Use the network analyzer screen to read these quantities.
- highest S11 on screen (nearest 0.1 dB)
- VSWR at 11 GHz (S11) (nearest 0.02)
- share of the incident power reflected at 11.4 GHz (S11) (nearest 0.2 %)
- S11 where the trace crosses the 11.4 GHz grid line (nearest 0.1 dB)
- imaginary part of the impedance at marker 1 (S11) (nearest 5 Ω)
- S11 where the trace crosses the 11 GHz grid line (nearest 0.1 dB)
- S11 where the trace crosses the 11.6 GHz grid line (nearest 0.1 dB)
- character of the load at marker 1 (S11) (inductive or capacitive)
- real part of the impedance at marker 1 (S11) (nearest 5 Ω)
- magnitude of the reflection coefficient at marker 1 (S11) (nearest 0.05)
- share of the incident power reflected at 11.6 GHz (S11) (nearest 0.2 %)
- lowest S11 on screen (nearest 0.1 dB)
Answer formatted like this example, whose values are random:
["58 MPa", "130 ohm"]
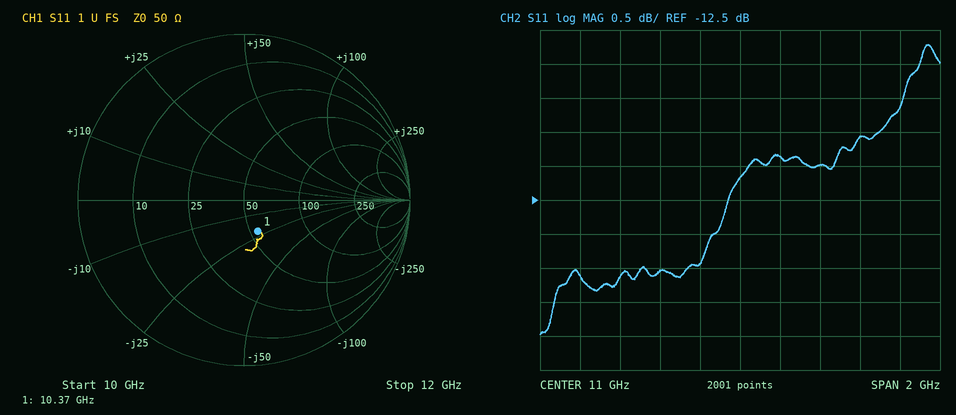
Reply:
["-10.2 dB", "1.66", "6.4 %", "-12.0 dB", "-20 Ω", "-12.2 dB", "-11.6 dB", "capacitive", "55 Ω", "0.20", "7.0 %", "-14.5 dB"]
